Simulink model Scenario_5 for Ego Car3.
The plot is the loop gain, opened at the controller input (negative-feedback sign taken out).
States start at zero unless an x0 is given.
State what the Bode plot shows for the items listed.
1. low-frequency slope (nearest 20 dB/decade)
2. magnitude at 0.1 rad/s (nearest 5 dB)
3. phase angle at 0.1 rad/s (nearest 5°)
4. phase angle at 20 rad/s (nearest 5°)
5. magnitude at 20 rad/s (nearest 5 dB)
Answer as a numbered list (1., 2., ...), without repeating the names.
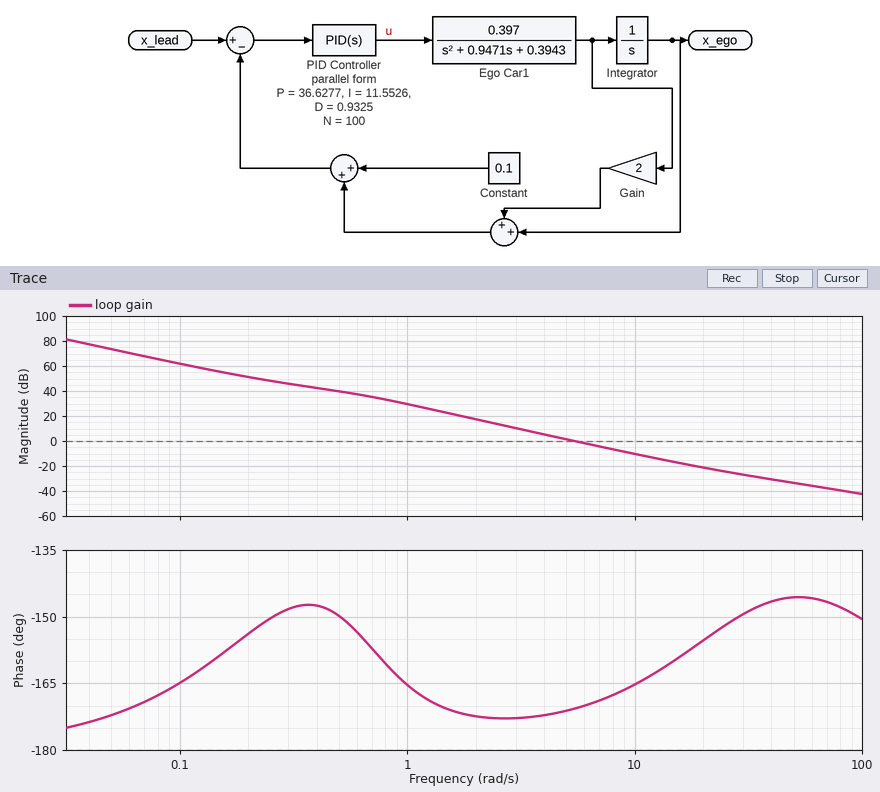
1. -40 dB/decade
2. 60 dB
3. -165°
4. -155°
5. -20 dB
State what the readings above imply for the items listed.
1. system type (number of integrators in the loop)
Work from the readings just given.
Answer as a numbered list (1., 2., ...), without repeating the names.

1. 2
